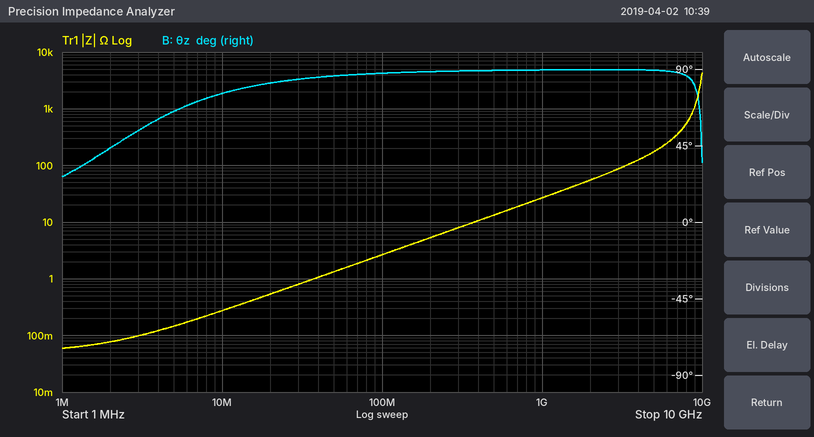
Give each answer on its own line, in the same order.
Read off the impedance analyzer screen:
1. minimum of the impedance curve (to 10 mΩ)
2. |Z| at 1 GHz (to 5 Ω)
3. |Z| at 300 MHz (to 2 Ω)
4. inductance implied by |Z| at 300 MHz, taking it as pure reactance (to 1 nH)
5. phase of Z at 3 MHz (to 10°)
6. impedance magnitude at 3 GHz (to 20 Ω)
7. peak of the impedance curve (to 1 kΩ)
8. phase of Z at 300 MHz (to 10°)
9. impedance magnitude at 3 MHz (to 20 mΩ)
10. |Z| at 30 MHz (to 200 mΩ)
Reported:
60 mΩ
25 Ω
8 Ω
4 nH
50°
80 Ω
4 kΩ
90°
100 mΩ
800 mΩ
